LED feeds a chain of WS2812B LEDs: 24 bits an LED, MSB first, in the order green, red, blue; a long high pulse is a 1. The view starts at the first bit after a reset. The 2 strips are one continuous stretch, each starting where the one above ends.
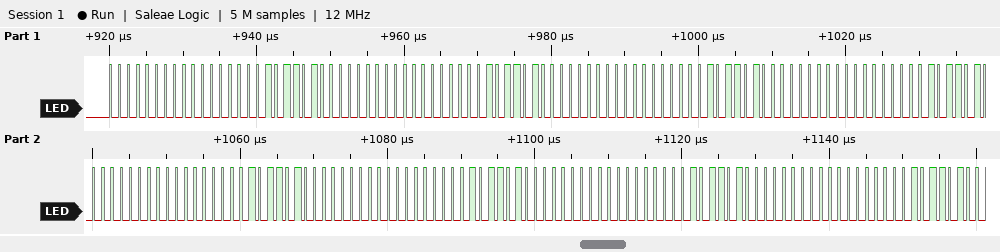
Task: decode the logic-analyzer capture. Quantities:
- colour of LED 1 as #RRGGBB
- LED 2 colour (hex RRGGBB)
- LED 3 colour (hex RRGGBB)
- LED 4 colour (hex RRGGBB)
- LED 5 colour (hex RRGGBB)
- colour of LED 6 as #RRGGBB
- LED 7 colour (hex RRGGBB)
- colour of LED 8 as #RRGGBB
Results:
#00005A
#00005A
#00005A
#00005A
#00005A
#00005A
#00005A
#00005A
